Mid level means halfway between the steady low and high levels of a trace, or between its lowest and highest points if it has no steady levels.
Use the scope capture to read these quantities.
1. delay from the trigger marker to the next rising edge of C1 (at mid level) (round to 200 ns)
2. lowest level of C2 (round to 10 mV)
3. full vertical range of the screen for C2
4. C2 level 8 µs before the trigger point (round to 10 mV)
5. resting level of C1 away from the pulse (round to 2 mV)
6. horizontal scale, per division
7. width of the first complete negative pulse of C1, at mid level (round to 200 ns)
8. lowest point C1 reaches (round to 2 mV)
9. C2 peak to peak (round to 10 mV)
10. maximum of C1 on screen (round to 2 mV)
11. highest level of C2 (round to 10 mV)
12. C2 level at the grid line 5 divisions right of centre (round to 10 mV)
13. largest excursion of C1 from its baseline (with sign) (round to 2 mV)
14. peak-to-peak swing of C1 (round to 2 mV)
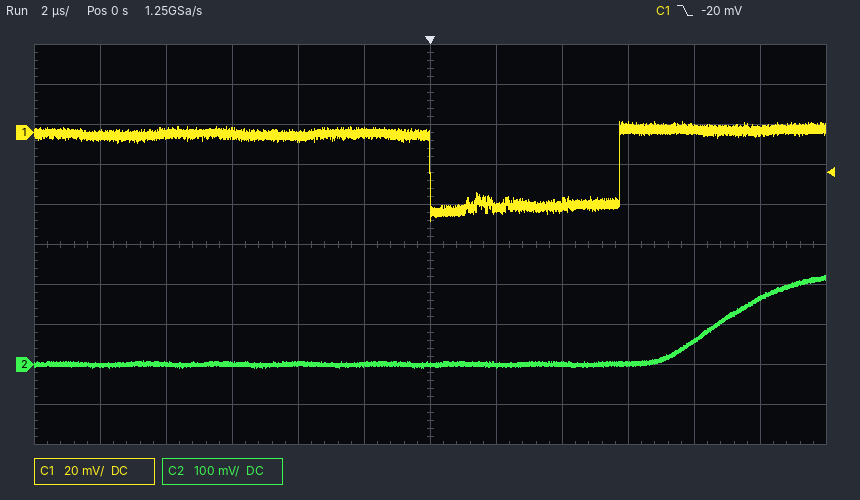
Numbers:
5.8 µs
-10 mV
1 V
0 mV
0 mV
2 µs
5.8 µs
-44 mV
230 mV
6 mV
220 mV
170 mV
-44 mV
50 mV
